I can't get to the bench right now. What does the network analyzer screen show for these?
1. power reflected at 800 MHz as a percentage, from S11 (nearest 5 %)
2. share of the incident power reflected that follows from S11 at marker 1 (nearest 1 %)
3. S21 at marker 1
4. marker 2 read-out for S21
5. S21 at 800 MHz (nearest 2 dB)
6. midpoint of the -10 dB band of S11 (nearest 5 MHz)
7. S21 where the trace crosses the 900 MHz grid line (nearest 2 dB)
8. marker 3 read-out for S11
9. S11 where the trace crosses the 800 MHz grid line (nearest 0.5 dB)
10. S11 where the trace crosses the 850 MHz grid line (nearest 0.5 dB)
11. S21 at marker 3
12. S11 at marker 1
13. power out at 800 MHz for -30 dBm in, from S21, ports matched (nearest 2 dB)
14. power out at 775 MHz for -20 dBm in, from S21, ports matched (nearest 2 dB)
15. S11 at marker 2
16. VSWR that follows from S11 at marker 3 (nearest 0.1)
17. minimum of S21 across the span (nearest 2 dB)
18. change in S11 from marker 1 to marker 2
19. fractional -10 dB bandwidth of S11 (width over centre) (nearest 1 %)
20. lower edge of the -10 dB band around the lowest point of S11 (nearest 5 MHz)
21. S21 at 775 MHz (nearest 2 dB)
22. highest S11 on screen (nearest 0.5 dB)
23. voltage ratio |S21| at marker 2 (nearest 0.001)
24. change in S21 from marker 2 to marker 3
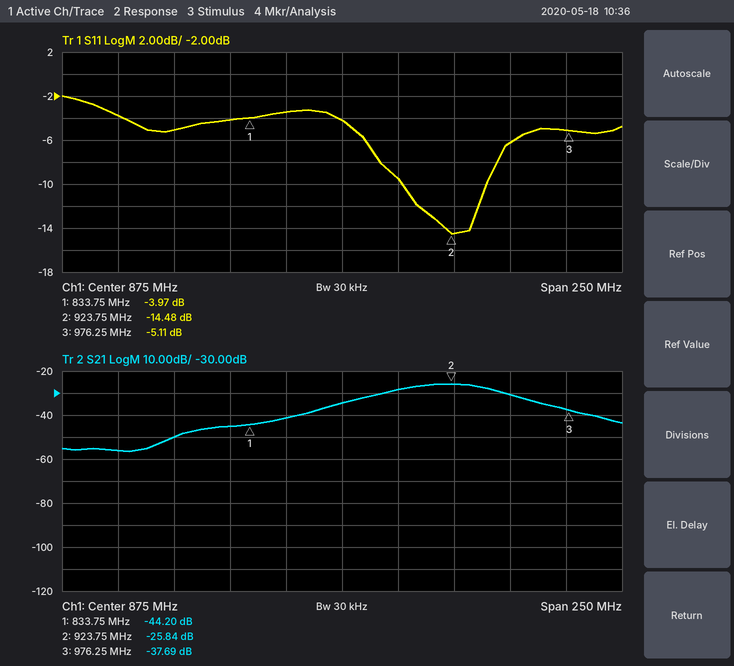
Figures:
30 %
40 %
-44.20 dB
-25.84 dB
-50 dB
920 MHz
-28 dB
-5.11 dB
-5.0 dB
-3.5 dB
-37.69 dB
-3.97 dB
-80 dBm
-76 dBm
-14.48 dB
3.5
-56 dB
-10.51 dB
4 %
900 MHz
-56 dB
-2.0 dB
0.051
-11.85 dB
